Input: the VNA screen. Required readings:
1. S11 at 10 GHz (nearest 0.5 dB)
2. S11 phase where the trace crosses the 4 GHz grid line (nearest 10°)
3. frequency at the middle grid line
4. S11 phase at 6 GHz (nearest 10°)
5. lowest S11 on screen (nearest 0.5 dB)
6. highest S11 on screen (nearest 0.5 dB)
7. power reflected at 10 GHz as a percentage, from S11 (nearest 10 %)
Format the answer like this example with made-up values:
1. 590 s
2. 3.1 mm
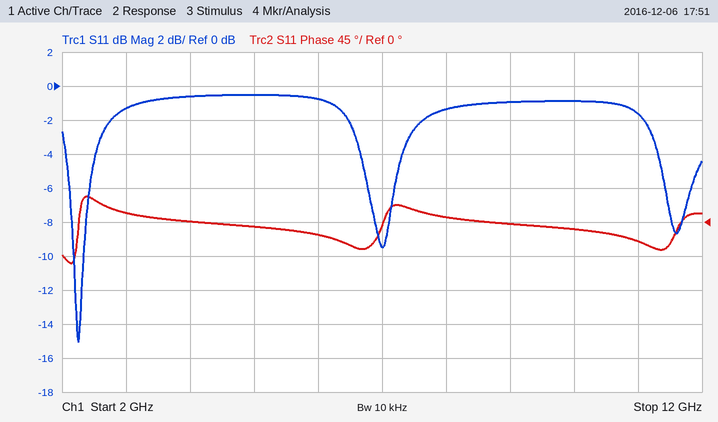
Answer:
1. -1.0 dB
2. 0°
3. 7 GHz
4. -20°
5. -15.0 dB
6. -0.5 dB
7. 80 %
